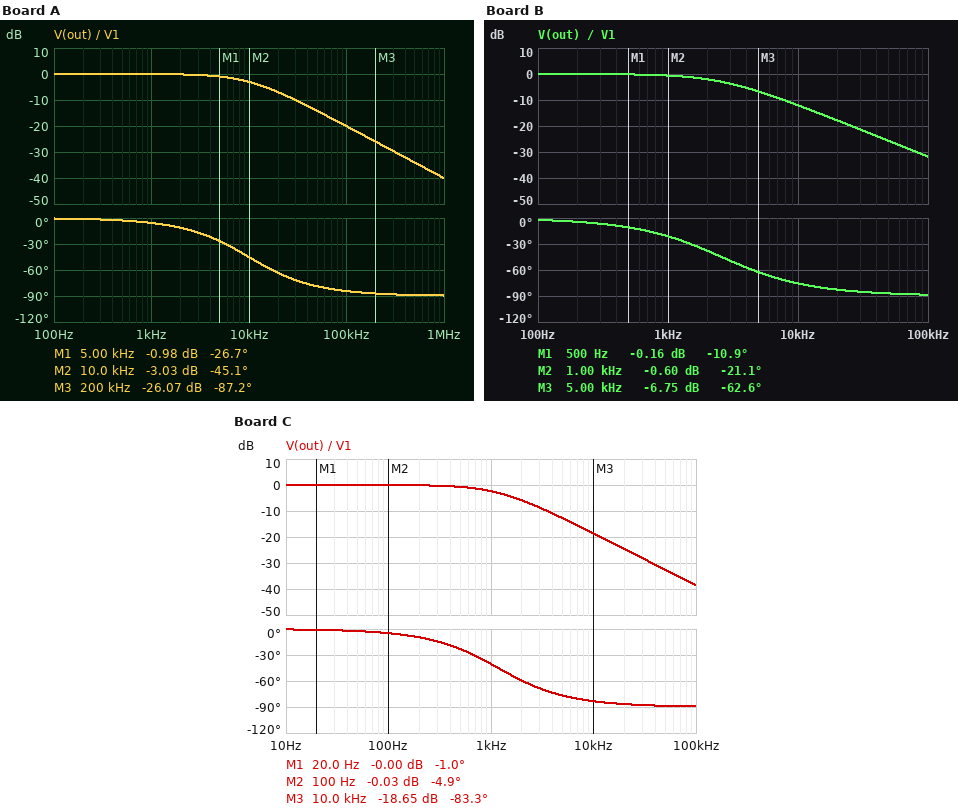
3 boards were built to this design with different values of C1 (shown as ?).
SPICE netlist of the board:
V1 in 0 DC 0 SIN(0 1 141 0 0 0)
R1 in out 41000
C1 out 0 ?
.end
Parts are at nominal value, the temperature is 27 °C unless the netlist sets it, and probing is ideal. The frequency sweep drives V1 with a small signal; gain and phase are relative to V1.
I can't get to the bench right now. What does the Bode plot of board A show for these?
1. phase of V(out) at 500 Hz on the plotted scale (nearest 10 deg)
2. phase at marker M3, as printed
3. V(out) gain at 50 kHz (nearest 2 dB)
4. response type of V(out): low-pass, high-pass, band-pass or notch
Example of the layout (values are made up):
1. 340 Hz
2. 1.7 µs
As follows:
1. 0 deg
2. -87.2 deg
3. -14 dB
4. low-pass
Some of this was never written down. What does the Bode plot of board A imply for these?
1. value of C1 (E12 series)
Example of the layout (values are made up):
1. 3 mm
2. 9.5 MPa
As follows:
1. 390 pF
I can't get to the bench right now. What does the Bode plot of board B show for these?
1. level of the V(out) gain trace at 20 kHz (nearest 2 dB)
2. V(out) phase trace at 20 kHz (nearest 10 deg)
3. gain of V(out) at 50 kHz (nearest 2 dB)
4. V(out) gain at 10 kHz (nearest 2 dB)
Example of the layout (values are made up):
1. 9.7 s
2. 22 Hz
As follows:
1. -18 dB
2. -80 deg
3. -26 dB
4. -12 dB
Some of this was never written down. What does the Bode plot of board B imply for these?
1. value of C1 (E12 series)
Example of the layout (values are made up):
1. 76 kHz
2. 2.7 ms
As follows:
1. 1.5 nF
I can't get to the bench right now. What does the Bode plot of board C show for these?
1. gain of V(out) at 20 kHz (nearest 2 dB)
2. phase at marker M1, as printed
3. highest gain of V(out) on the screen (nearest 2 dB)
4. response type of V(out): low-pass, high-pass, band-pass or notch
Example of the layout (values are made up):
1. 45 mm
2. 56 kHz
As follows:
1. -24 dB
2. -1.0 deg
3. 0 dB
4. low-pass
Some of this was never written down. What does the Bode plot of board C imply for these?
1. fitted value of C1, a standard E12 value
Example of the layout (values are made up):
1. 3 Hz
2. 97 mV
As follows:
1. 3.3 nF
